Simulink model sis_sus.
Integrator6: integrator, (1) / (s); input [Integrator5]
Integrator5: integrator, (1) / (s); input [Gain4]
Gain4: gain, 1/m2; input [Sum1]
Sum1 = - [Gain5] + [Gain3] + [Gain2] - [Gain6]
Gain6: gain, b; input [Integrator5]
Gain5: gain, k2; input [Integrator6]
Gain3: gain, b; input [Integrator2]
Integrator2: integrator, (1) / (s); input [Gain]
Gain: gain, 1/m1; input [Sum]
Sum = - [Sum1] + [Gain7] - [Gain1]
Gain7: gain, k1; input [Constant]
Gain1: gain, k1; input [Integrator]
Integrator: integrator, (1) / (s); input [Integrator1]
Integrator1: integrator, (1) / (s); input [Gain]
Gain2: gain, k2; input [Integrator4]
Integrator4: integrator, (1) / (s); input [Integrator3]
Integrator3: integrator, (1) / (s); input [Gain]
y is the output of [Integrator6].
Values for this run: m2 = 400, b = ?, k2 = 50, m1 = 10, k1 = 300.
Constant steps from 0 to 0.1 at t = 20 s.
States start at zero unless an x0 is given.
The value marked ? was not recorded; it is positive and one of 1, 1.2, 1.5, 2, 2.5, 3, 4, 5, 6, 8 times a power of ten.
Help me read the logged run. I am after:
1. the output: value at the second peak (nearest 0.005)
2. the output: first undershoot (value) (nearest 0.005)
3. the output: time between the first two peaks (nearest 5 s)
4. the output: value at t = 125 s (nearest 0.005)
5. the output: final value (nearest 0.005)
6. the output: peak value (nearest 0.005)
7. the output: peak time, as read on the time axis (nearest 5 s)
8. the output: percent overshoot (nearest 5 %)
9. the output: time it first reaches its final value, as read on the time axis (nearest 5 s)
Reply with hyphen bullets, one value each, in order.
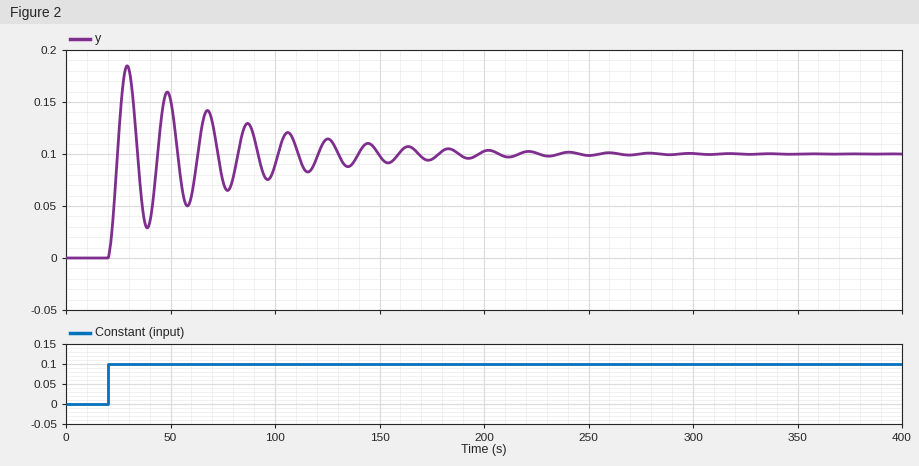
- 0.160
- 0.030
- 20 s
- 0.115
- 0.100
- 0.185
- 30 s
- 85 %
- 25 s
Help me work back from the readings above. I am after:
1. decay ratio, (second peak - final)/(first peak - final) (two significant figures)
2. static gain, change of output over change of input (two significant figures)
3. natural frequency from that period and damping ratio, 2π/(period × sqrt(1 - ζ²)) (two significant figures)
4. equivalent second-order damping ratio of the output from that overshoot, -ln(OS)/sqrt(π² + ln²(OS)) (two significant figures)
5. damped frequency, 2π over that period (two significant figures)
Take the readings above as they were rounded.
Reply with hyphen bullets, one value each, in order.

- 0.71
- 1.0
- 0.31 rad/s
- 0.052
- 0.31 rad/s
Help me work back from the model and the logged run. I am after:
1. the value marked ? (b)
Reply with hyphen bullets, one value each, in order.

- 20
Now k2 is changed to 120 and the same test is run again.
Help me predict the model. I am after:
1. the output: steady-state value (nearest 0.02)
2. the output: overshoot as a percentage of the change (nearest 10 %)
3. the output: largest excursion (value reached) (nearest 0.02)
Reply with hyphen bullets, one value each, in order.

- 0.10
- 90 %
- 0.20
